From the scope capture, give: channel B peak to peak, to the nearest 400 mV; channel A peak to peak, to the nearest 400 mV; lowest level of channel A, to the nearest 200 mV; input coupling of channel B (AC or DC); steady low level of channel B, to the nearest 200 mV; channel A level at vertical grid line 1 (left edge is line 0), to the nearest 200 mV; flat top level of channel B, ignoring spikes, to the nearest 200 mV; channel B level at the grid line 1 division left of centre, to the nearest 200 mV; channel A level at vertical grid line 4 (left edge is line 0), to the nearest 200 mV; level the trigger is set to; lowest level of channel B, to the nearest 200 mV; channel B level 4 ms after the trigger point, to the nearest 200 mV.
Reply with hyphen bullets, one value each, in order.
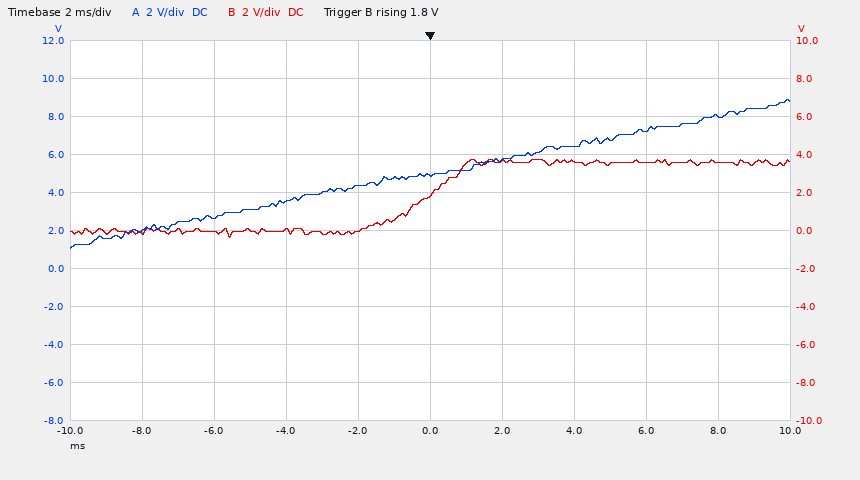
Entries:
- 4.0 V
- 8.0 V
- 1.0 V
- DC
- 0.0 V
- 2.0 V
- 3.6 V
- 0.0 V
- 4.4 V
- 1.8 V
- -400 mV
- 3.6 V
